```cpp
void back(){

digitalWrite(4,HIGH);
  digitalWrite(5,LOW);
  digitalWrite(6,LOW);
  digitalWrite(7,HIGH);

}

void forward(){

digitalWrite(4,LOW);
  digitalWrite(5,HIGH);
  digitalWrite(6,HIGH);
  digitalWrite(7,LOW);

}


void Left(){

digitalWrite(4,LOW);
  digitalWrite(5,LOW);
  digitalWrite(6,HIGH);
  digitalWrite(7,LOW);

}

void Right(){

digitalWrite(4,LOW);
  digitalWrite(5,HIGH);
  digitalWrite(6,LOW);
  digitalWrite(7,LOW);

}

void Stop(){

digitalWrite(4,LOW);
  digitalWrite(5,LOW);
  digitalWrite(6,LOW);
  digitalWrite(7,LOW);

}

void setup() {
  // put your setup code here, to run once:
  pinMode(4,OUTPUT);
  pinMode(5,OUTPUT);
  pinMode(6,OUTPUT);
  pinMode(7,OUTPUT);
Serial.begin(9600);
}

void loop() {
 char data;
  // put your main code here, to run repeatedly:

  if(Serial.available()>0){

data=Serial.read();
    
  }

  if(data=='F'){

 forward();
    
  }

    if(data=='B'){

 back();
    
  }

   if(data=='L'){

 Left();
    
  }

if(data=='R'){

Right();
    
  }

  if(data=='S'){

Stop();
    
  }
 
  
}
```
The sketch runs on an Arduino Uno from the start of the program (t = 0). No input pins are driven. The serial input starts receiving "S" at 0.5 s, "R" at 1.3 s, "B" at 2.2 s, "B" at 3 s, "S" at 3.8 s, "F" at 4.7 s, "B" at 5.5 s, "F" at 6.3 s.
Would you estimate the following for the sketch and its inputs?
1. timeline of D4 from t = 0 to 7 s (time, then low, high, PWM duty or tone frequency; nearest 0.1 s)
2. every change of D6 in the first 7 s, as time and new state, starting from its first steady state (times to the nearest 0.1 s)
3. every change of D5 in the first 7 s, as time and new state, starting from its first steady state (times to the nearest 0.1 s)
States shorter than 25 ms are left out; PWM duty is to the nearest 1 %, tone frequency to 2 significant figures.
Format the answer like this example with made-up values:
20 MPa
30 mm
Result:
0 s low; 2.2 s high; 3.8 s low; 5.5 s high; 6.3 s low
0 s low; 4.7 s high; 5.5 s low; 6.3 s high
0 s low; 1.3 s high; 2.2 s low; 4.7 s high; 5.5 s low; 6.3 s high
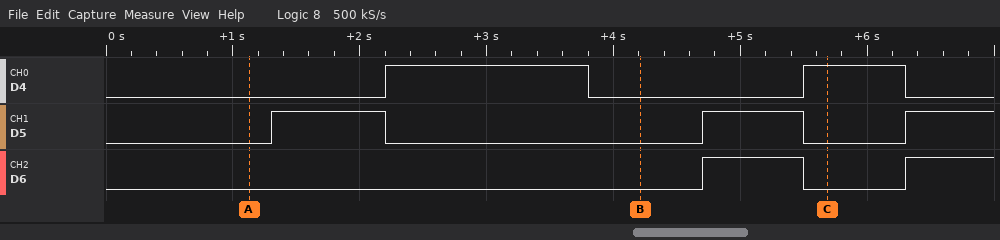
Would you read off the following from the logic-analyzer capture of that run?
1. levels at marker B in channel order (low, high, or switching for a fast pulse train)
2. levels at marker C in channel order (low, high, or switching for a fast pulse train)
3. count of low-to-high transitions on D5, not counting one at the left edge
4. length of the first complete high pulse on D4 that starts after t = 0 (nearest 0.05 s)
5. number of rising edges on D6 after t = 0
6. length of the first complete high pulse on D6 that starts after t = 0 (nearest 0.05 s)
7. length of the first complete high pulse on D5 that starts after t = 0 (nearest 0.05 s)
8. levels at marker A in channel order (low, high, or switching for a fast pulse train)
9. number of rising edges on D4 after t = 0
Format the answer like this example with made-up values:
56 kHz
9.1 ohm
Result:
D4 low, D5 low, D6 low
D4 high, D5 low, D6 low
3
1.60 s
2
0.80 s
0.90 s
D4 low, D5 low, D6 low
2
